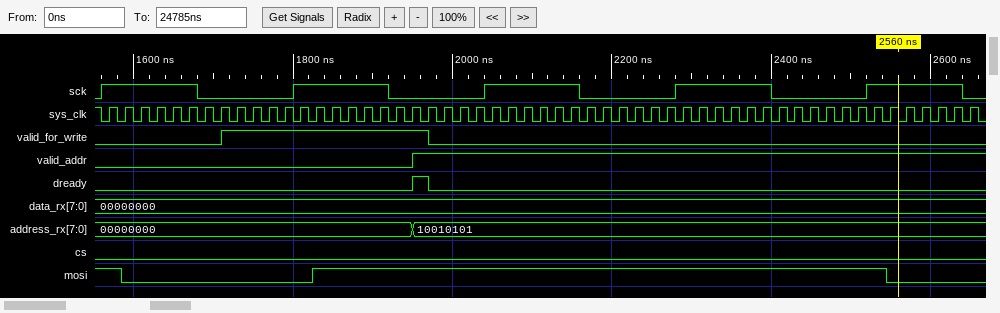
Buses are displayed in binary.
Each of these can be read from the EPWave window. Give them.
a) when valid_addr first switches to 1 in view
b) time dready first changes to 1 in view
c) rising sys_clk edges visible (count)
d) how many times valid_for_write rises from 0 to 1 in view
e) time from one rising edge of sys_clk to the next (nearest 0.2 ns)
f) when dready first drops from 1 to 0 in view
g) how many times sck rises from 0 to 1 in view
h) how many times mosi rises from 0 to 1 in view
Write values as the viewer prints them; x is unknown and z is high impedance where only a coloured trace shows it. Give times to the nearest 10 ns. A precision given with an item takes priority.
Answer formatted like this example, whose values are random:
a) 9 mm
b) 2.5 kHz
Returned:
a) 1950 ns
b) 1950 ns
c) 55
d) 1
e) 20 ns
f) 1970 ns
g) 5
h) 1
